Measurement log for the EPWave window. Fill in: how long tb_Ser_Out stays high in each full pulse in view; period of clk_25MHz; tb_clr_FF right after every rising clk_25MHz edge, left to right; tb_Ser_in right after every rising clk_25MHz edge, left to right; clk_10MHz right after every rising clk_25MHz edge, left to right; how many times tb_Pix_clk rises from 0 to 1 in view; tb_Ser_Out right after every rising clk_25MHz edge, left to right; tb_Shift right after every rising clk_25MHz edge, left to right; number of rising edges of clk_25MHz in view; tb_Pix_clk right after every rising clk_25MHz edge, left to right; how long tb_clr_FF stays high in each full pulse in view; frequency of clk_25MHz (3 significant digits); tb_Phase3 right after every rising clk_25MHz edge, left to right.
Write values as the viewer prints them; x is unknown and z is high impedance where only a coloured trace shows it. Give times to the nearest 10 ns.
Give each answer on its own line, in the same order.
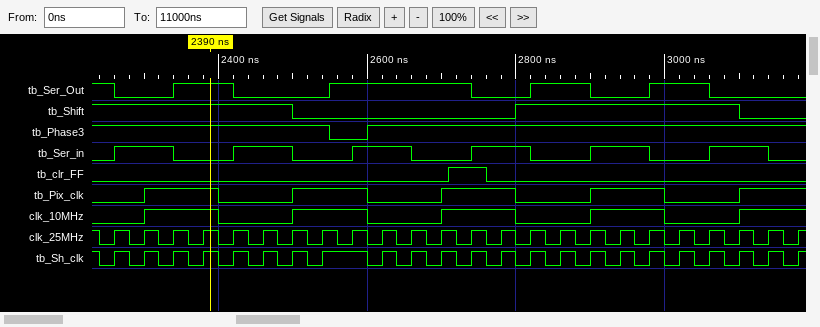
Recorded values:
80 ns, 190 ns, 80 ns, 80 ns
40 ns
0 0 0 0 0 0 0 0 0 0 0 0 1 0 0 0 0 0 0 0 0 0 0 0
1 1 0 0 1 1 0 0 1 1 0 0 1 1 0 0 1 1 0 0 1 1 0 0
0 1 1 1 0 0 1 1 1 0 0 1 1 1 0 0 1 1 1 0 0 1 1 1
5
0 0 1 1 0 0 0 0 1 1 1 1 0 0 1 1 0 0 1 1 0 0 0 0
1 1 1 1 1 1 0 0 0 0 0 0 0 0 1 1 1 1 1 1 1 0 0 0
24
0 1 1 1 0 0 1 1 1 0 0 1 1 1 0 0 1 1 1 0 0 1 1 1
50 ns
25.0 MHz
1 1 1 1 1 1 1 1 0 1 1 1 1 1 1 1 1 1 1 1 1 1 1 1
